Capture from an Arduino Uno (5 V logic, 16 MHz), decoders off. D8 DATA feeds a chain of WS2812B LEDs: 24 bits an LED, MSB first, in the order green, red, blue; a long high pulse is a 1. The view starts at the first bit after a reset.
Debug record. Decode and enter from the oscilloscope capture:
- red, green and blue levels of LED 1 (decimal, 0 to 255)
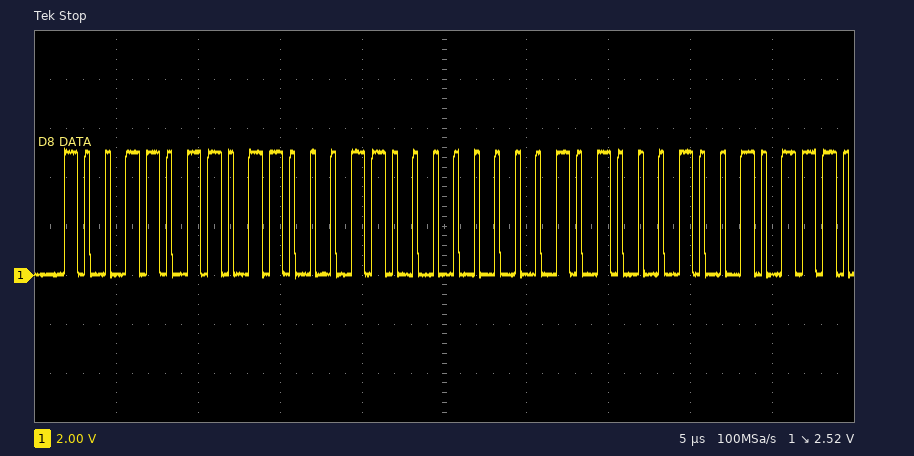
99, 155, 0
